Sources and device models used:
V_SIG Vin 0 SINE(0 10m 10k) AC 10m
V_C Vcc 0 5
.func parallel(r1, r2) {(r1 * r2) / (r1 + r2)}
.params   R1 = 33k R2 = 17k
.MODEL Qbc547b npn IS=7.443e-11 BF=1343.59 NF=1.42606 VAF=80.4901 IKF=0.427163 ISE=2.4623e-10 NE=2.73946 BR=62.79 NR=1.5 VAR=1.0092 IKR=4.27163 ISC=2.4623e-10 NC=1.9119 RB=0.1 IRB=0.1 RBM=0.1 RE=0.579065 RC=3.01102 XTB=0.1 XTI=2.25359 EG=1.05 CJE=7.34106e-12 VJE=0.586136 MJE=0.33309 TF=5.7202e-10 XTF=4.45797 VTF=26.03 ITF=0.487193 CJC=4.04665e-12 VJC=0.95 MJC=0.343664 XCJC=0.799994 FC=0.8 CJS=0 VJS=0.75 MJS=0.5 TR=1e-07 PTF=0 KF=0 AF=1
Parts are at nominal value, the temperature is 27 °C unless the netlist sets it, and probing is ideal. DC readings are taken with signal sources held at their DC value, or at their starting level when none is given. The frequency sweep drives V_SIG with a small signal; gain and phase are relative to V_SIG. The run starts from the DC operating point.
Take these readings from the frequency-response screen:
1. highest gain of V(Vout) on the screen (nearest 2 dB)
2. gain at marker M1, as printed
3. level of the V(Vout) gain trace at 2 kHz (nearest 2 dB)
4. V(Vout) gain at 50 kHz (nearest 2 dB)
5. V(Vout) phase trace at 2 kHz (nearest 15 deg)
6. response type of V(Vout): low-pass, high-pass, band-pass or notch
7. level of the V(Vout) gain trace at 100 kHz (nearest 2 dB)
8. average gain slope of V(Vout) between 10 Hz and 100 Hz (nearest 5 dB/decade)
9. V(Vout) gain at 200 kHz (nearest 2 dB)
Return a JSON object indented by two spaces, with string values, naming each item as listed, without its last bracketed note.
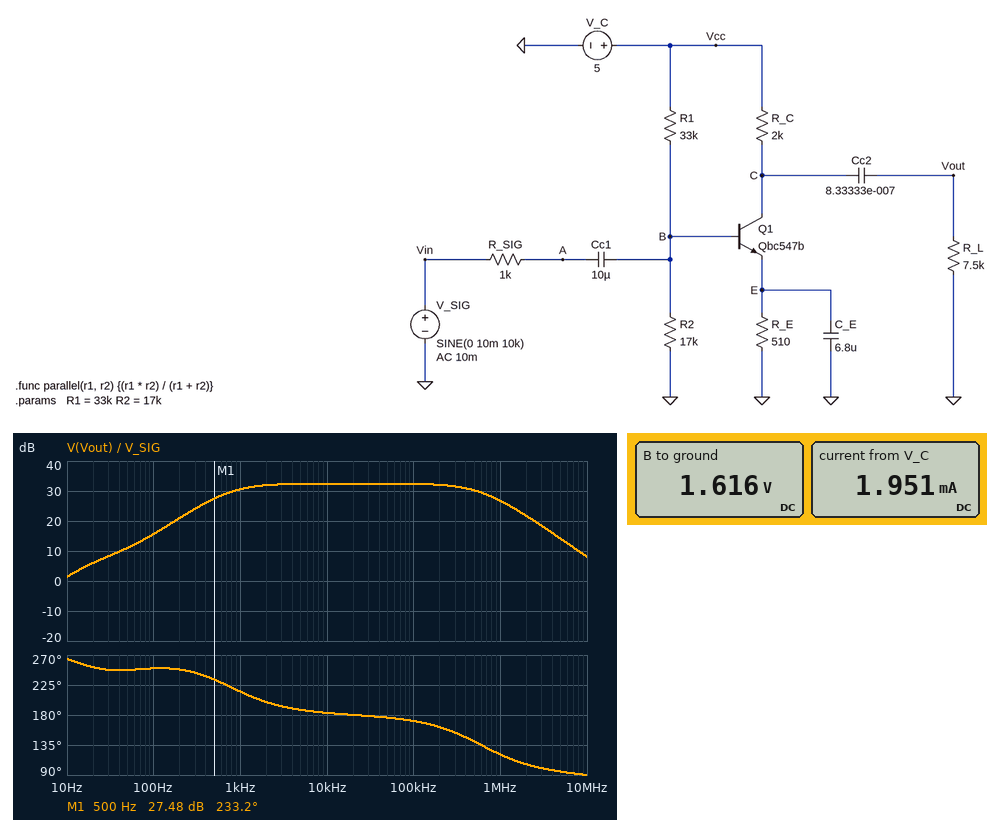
{
  "highest gain of V(Vout) on the screen": "32 dB",
  "gain at marker M1, as printed": "27.48 dB",
  "level of the V(Vout) gain trace at 2 kHz": "32 dB",
  "V(Vout) gain at 50 kHz": "32 dB",
  "V(Vout) phase trace at 2 kHz": "195 deg",
  "response type of V(Vout): low-pass, high-pass, band-pass or notch": "band-pass",
  "level of the V(Vout) gain trace at 100 kHz": "32 dB",
  "average gain slope of V(Vout) between 10 Hz and 100 Hz": "15 dB/decade",
  "V(Vout) gain at 200 kHz": "32 dB"
}
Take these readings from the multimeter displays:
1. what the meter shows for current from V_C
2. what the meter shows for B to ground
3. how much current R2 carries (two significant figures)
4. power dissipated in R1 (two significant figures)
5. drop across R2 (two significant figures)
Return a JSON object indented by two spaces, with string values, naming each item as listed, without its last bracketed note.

{
  "what the meter shows for current from V_C": "1.951 mA",
  "what the meter shows for B to ground": "1.616 V",
  "how much current R2 carries": "95 µA",
  "power dissipated in R1": "350 µW",
  "drop across R2": "1.6 V"
}
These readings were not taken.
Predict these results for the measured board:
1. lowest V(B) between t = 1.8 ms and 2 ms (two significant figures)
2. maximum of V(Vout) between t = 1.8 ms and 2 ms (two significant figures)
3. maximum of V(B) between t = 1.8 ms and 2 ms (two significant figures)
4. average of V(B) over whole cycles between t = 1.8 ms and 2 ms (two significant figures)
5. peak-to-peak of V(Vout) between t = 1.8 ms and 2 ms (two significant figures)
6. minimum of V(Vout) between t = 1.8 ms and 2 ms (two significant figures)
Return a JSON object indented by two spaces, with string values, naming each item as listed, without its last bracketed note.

{
  "lowest V(B) between t = 1.8 ms and 2 ms": "1.6 V",
  "maximum of V(Vout) between t = 1.8 ms and 2 ms": "350 mV",
  "maximum of V(B) between t = 1.8 ms and 2 ms": "1.6 V",
  "average of V(B) over whole cycles between t = 1.8 ms and 2 ms": "1.6 V",
  "peak-to-peak of V(Vout) between t = 1.8 ms and 2 ms": "550 mV",
  "minimum of V(Vout) between t = 1.8 ms and 2 ms": "-200 mV"
}
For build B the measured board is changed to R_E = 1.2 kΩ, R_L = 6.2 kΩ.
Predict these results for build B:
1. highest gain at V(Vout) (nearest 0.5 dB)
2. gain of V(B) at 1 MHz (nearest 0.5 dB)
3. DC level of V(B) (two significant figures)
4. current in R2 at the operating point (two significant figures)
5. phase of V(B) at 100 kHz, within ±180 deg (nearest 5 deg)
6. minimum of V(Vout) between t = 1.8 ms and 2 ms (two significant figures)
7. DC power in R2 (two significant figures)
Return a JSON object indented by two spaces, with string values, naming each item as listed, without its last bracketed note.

{
  "highest gain at V(Vout)": "28.0 dB",
  "gain of V(B) at 1 MHz": "-3.0 dB",
  "DC level of V(B)": "1.7 V",
  "current in R2 at the operating point": "98 µA",
  "phase of V(B) at 100 kHz, within ±180 deg": "-5 deg",
  "minimum of V(Vout) between t = 1.8 ms and 2 ms": "-270 mV",
  "DC power in R2": "160 µW"
}
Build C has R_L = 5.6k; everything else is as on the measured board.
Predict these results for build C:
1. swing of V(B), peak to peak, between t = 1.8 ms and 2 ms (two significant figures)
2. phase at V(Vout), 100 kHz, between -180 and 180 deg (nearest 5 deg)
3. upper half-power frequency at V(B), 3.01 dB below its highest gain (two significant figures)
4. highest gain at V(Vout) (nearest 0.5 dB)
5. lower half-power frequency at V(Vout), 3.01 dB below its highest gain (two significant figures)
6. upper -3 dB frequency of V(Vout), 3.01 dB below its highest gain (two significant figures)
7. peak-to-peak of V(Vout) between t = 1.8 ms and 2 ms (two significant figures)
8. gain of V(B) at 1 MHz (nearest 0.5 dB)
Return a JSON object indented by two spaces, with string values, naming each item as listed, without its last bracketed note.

{
  "swing of V(B), peak to peak, between t = 1.8 ms and 2 ms": "10 mV",
  "phase at V(Vout), 100 kHz, between -180 and 180 deg": "170 deg",
  "upper half-power frequency at V(B), 3.01 dB below its highest gain": "300 kHz",
  "highest gain at V(Vout)": "32.0 dB",
  "lower half-power frequency at V(Vout), 3.01 dB below its highest gain": "750 Hz",
  "upper -3 dB frequency of V(Vout), 3.01 dB below its highest gain": "630 kHz",
  "peak-to-peak of V(Vout) between t = 1.8 ms and 2 ms": "530 mV",
  "gain of V(B) at 1 MHz": "-8.5 dB"
}
